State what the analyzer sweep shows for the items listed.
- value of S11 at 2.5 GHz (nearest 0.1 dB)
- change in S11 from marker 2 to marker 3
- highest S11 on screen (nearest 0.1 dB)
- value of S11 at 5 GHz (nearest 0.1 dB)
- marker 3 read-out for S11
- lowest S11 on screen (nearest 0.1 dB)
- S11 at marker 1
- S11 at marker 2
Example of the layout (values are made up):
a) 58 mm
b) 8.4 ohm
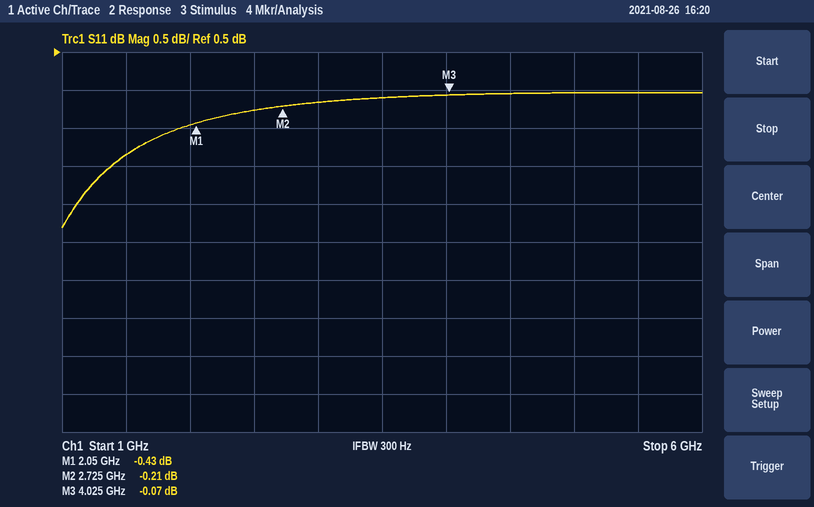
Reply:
a) -0.3 dB
b) 0.14 dB
c) 0.0 dB
d) 0.0 dB
e) -0.07 dB
f) -1.8 dB
g) -0.43 dB
h) -0.21 dB
